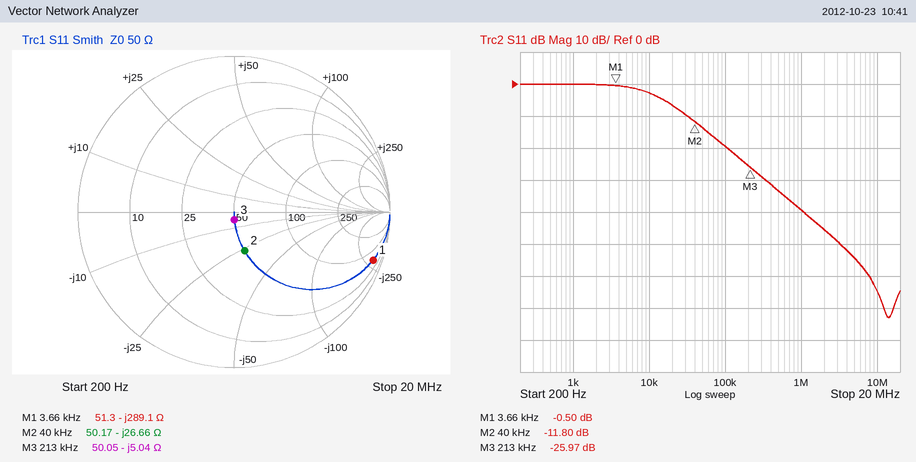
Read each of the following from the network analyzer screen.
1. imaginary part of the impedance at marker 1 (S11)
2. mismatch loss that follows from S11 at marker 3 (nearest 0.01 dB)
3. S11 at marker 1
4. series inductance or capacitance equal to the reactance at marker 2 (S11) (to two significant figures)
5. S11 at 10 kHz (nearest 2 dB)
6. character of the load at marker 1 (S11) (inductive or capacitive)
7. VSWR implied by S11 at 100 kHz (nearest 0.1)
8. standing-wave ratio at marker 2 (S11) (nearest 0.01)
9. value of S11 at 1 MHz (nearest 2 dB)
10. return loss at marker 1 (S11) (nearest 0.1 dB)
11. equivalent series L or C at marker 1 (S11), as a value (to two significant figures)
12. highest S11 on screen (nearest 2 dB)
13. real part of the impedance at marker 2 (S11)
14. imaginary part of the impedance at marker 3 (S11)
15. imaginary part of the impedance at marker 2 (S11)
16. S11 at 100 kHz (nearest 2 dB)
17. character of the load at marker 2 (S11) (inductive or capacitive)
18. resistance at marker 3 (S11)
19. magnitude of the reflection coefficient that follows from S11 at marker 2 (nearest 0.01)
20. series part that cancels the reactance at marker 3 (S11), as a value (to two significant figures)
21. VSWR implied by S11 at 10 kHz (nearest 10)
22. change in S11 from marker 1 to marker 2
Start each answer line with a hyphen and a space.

- -289.1 Ω
- 0.01 dB
- -0.50 dB
- 150 nF
- -2 dB
- capacitive
- 1.2
- 1.69
- -40 dB
- 0.5 dB
- 150 nF
- 0 dB
- 50.17 Ω
- -5.04 Ω
- -26.66 Ω
- -20 dB
- capacitive
- 50.05 Ω
- 0.26
- 3.8 µH
- 10
- -11.30 dB
